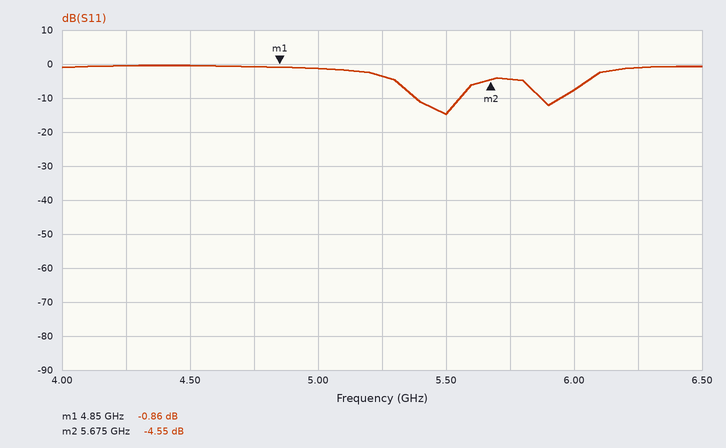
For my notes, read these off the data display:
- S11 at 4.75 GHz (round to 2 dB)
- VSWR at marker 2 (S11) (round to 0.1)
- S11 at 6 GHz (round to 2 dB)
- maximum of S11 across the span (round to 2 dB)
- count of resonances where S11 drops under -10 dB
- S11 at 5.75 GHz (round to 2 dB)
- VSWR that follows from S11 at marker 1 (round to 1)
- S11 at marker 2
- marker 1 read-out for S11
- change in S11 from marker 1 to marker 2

0 dB
3.9
-8 dB
0 dB
2
-4 dB
20
-4.55 dB
-0.86 dB
-3.69 dB
